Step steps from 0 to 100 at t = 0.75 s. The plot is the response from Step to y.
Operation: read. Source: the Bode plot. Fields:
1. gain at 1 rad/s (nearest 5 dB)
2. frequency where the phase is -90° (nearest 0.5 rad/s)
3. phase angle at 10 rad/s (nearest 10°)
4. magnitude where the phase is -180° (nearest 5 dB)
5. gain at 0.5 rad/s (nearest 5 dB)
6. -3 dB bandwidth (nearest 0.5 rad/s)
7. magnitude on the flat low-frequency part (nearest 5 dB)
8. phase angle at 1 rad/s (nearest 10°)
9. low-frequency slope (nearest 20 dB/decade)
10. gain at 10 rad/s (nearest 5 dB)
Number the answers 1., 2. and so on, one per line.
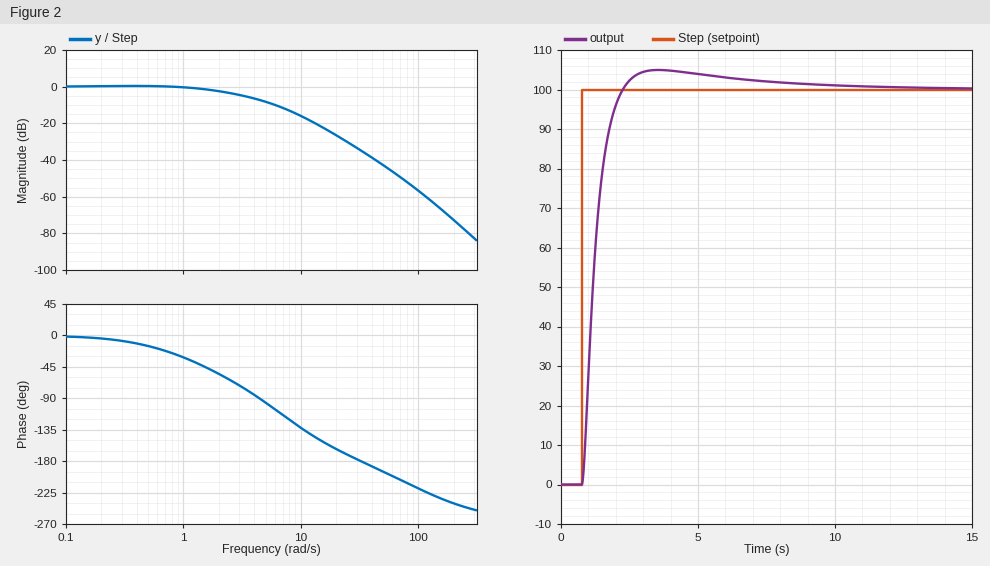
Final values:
1. 0 dB
2. 4.5 rad/s
3. -130°
4. -35 dB
5. 0 dB
6. 2.0 rad/s
7. 0 dB
8. -30°
9. 0 dB/decade
10. -15 dB
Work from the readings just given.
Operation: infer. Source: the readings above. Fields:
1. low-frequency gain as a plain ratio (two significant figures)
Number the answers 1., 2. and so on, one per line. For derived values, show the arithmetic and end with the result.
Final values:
1. 10^(0 / 20) = 1.0
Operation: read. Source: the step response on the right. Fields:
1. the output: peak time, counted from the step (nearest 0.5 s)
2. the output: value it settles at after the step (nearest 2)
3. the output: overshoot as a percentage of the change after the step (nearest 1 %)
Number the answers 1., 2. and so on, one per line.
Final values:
1. 3.0 s
2. 100
3. 5 %
